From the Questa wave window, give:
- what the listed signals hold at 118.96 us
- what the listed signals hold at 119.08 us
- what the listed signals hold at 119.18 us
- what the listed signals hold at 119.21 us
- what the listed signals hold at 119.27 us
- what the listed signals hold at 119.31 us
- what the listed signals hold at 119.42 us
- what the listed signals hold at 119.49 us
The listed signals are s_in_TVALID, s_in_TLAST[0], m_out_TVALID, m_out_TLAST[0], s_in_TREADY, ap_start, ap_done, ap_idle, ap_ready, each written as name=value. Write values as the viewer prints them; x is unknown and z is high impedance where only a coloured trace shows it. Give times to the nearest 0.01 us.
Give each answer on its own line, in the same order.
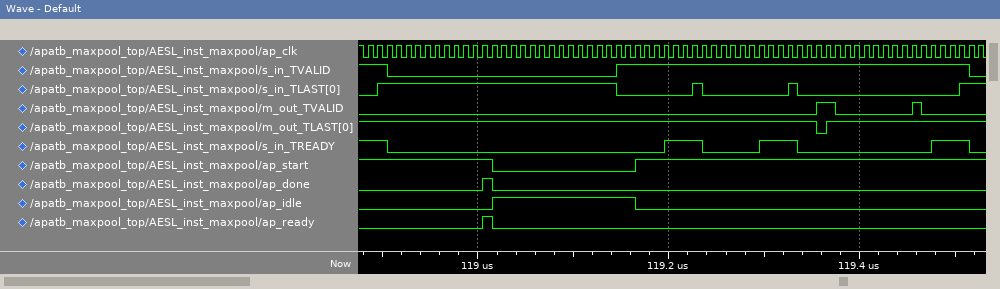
s_in_TVALID=0, s_in_TLAST[0]=1, m_out_TVALID=0, m_out_TLAST[0]=1, s_in_TREADY=0, ap_start=1, ap_done=0, ap_idle=0, ap_ready=0
s_in_TVALID=0, s_in_TLAST[0]=1, m_out_TVALID=0, m_out_TLAST[0]=1, s_in_TREADY=0, ap_start=0, ap_done=0, ap_idle=1, ap_ready=0
s_in_TVALID=1, s_in_TLAST[0]=0, m_out_TVALID=0, m_out_TLAST[0]=1, s_in_TREADY=0, ap_start=1, ap_done=0, ap_idle=0, ap_ready=0
s_in_TVALID=1, s_in_TLAST[0]=0, m_out_TVALID=0, m_out_TLAST[0]=1, s_in_TREADY=1, ap_start=1, ap_done=0, ap_idle=0, ap_ready=0
s_in_TVALID=1, s_in_TLAST[0]=0, m_out_TVALID=0, m_out_TLAST[0]=1, s_in_TREADY=0, ap_start=1, ap_done=0, ap_idle=0, ap_ready=0
s_in_TVALID=1, s_in_TLAST[0]=0, m_out_TVALID=0, m_out_TLAST[0]=1, s_in_TREADY=1, ap_start=1, ap_done=0, ap_idle=0, ap_ready=0
s_in_TVALID=1, s_in_TLAST[0]=0, m_out_TVALID=0, m_out_TLAST[0]=1, s_in_TREADY=0, ap_start=1, ap_done=0, ap_idle=0, ap_ready=0
s_in_TVALID=1, s_in_TLAST[0]=0, m_out_TVALID=0, m_out_TLAST[0]=1, s_in_TREADY=1, ap_start=1, ap_done=0, ap_idle=0, ap_ready=0
